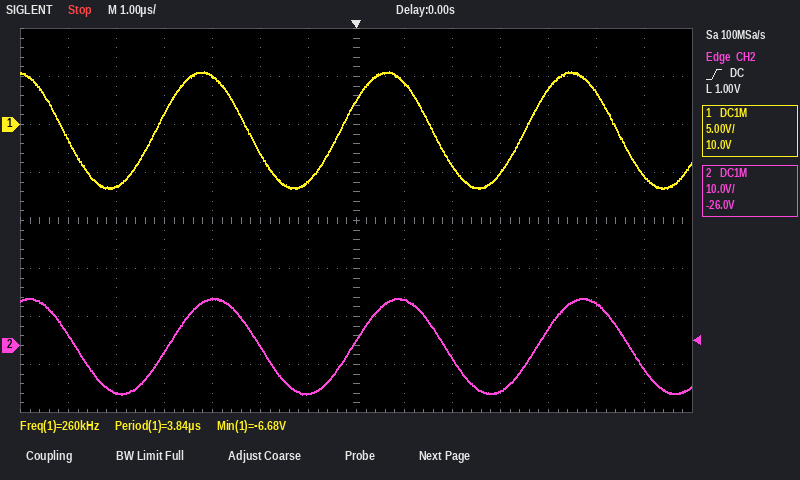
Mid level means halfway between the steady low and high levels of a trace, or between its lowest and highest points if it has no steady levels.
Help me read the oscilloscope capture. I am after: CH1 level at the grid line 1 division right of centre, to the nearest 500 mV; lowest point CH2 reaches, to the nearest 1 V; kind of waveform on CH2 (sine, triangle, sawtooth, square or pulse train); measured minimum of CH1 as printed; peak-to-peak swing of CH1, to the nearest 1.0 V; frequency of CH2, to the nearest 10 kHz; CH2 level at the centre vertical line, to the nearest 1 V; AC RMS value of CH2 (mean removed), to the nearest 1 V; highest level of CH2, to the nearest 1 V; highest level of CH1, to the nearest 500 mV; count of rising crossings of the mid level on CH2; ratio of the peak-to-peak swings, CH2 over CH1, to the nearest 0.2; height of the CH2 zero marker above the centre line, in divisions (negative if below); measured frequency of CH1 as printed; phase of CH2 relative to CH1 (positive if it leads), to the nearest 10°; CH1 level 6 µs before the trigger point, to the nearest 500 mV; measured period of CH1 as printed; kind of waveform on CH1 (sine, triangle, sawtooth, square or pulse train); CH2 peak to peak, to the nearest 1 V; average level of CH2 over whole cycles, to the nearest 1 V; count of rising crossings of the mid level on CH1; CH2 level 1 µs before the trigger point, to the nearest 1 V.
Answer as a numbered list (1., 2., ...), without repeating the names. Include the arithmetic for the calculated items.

1. 4.5 V
2. -10 V
3. sine
4. -6.68 V
5. 12.0 V
6. 260 kHz
7. 1 V
8. 20 V / (2√2) ≈ 7 V
9. 10 V
10. 5.5 V
11. 3
12. 20 V / 12.0 V ≈ 1.67, so 1.6 to the nearest 0.2
13. -2.6 div
14. 260 kHz
15. -20°
16. -1.5 V
17. 3.84 µs
18. sine
19. 10 V − (-10 V) = 20 V
20. (10 V + (-10 V)) / 2 ≈ 0 V
21. 3
22. -10 V
